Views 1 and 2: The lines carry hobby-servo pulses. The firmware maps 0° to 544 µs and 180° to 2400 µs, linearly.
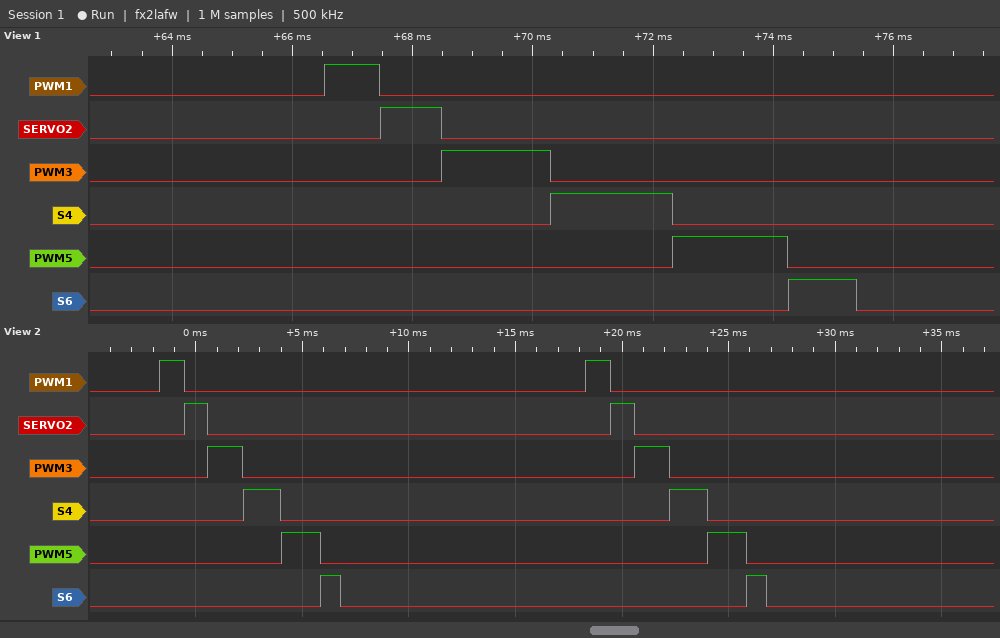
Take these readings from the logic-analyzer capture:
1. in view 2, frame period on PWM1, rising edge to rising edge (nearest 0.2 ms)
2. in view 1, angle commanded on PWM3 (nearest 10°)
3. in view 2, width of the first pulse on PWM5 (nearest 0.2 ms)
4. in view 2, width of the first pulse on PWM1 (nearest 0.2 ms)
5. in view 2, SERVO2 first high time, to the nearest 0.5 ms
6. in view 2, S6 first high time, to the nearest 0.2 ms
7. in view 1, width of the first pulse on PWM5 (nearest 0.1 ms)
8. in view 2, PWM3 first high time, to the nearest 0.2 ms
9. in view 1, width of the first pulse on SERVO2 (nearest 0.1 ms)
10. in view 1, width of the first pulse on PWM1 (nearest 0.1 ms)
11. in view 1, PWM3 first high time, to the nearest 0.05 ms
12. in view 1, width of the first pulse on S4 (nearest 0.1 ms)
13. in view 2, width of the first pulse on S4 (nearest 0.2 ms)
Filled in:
20.0 ms
120°
1.8 ms
1.2 ms
1.0 ms
1.0 ms
1.9 ms
1.6 ms
1.0 ms
0.9 ms
1.80 ms
2.0 ms
1.8 ms
